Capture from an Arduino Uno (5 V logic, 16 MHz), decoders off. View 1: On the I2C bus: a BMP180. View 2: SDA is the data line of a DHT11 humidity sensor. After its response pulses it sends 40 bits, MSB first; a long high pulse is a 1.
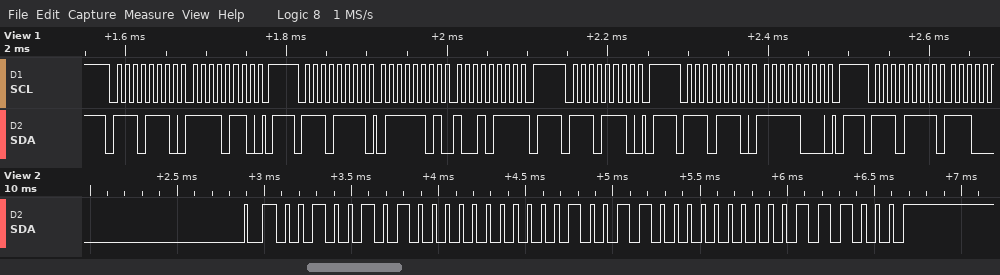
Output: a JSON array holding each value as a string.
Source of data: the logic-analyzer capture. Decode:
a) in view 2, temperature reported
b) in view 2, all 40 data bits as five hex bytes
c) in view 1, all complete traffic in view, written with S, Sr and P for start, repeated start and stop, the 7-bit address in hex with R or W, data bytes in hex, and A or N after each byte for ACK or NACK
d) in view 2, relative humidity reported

["19.0 °C", "25 00 13 00 38", "S 77W A F6 A P S 77R A 7D A 97 N P S 77W A P S 77W A F8 A P S 77R A", "37 %"]
